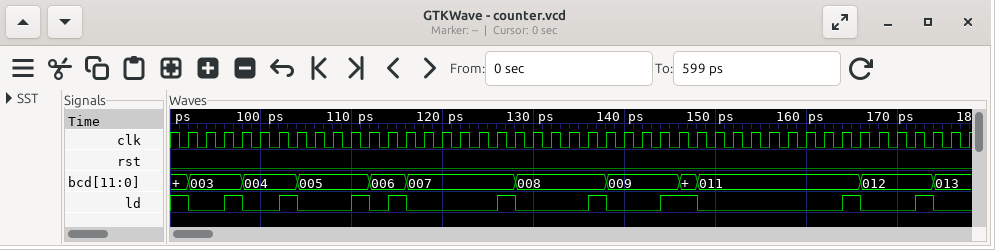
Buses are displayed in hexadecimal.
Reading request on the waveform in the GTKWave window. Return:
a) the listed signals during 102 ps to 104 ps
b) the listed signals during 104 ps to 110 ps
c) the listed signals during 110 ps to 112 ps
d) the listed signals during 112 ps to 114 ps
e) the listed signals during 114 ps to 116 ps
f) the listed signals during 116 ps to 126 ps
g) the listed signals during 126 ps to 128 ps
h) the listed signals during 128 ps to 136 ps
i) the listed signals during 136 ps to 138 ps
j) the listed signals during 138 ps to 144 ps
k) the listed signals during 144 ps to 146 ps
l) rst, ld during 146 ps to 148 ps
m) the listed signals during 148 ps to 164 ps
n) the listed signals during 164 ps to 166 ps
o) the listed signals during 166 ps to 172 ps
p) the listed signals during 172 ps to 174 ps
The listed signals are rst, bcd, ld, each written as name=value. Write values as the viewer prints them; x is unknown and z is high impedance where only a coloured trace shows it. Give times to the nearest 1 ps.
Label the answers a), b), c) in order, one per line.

a) rst=0, bcd=004, ld=1
b) rst=0, bcd=005, ld=0
c) rst=0, bcd=005, ld=1
d) rst=0, bcd=006, ld=0
e) rst=0, bcd=006, ld=1
f) rst=0, bcd=007, ld=0
g) rst=0, bcd=007, ld=1
h) rst=0, bcd=008, ld=0
i) rst=0, bcd=008, ld=1
j) rst=0, bcd=009, ld=0
k) rst=0, bcd=009, ld=1
l) rst=0, ld=1
m) rst=0, bcd=011, ld=0
n) rst=0, bcd=011, ld=1
o) rst=0, bcd=012, ld=0
p) rst=0, bcd=012, ld=1
